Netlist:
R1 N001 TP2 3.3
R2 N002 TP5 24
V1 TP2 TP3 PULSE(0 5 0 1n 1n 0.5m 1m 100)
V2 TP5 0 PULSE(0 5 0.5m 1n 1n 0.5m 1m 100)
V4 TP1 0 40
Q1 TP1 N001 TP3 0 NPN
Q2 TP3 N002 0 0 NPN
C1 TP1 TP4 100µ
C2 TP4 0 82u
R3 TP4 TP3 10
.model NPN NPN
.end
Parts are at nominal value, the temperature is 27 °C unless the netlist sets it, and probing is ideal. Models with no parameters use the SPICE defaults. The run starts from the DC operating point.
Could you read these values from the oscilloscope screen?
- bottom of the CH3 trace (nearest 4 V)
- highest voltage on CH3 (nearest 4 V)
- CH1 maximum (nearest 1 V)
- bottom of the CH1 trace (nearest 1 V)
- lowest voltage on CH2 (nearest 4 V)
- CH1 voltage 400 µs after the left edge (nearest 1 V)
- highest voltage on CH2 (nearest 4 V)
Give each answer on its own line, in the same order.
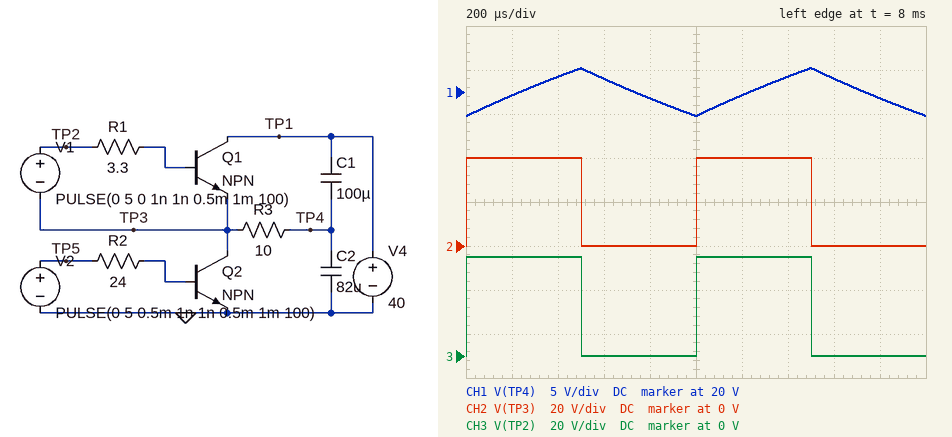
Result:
0 V
44 V
23 V
17 V
0 V
22 V
40 V
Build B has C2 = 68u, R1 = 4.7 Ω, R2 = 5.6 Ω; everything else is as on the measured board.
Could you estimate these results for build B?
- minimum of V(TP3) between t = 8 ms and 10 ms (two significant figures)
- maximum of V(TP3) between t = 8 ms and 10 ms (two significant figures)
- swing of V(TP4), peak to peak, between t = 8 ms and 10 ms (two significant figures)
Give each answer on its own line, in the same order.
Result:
39 mV
40 V
5.9 V
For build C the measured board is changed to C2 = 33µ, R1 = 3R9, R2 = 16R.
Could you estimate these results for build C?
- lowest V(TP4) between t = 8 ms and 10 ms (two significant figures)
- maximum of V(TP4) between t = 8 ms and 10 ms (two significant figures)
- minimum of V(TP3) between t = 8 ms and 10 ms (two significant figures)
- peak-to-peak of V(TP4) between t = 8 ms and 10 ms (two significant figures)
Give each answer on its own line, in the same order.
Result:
16 V
24 V
57 mV
7.4 V
